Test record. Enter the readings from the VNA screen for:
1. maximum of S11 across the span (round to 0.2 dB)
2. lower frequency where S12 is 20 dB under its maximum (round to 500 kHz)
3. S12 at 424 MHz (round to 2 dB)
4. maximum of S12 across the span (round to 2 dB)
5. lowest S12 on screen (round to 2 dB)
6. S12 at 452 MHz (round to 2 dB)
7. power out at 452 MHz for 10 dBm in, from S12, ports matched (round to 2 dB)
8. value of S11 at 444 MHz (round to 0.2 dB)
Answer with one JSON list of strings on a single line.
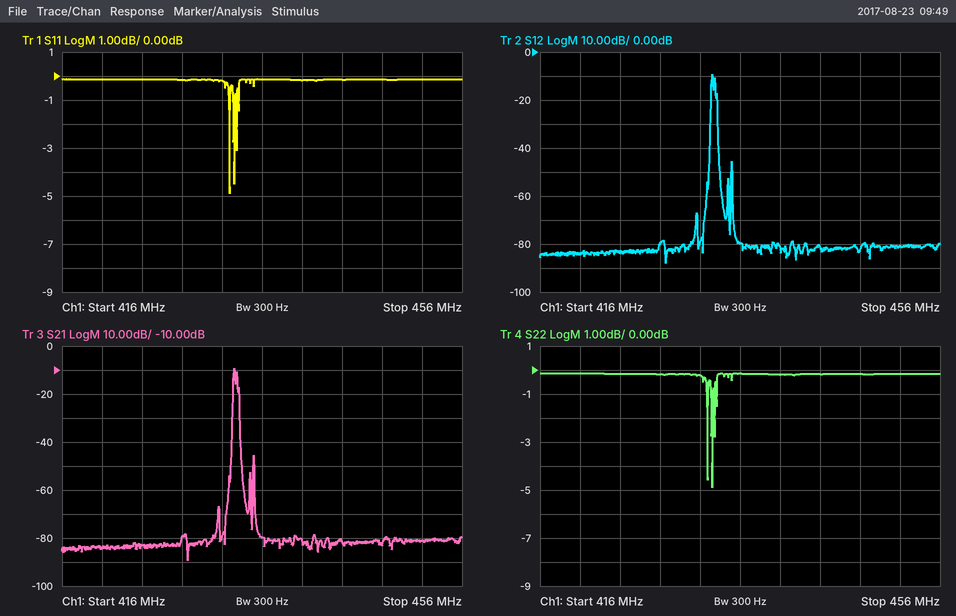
["-0.2 dB", "433.0 MHz", "-84 dB", "-10 dB", "-88 dB", "-80 dB", "-70 dBm", "-0.2 dB"]
